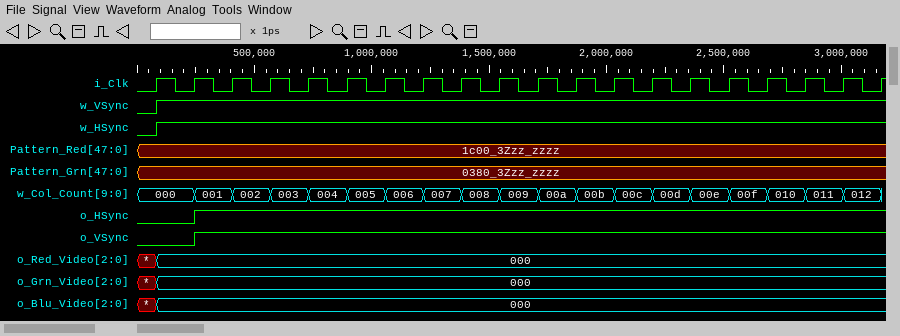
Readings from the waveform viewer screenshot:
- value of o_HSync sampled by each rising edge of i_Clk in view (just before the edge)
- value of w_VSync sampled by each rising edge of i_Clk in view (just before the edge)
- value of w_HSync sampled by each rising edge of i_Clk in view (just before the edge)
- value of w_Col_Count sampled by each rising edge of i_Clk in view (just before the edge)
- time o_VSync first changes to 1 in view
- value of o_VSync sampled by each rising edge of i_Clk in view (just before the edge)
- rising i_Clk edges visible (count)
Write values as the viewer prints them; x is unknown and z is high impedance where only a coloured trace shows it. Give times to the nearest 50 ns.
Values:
0 0 1 1 1 1 1 1 1 1 1 1 1 1 1 1 1 1 1 1
0 1 1 1 1 1 1 1 1 1 1 1 1 1 1 1 1 1 1 1
0 1 1 1 1 1 1 1 1 1 1 1 1 1 1 1 1 1 1 1
000, 000, 001, 002, 003, 004, 005, 006, 007, 008, 009, 00a, 00b, 00c, 00d, 00e, 00f, 010, 011, 012
250 ns
0 0 1 1 1 1 1 1 1 1 1 1 1 1 1 1 1 1 1 1
20
